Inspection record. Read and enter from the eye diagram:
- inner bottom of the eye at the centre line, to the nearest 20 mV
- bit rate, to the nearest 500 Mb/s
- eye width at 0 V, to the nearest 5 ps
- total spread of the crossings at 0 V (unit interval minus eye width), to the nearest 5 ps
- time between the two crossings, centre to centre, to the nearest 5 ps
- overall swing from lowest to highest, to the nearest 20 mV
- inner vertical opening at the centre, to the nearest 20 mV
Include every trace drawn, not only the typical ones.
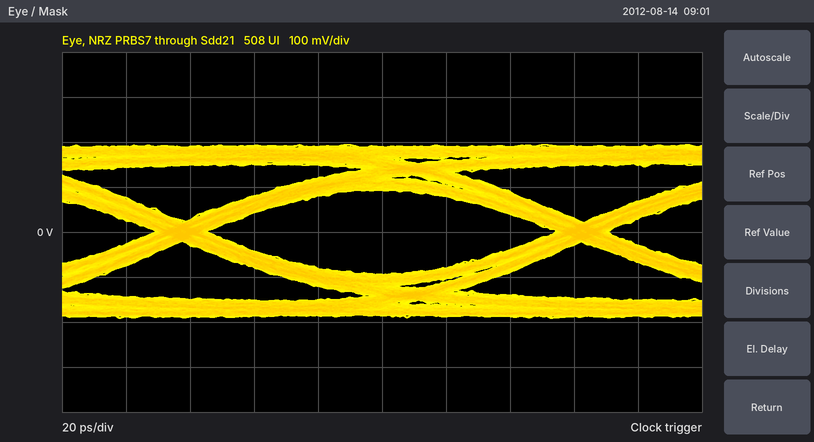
-100 mV
8.0 Gb/s
110 ps
15 ps
125 ps
380 mV
180 mV
